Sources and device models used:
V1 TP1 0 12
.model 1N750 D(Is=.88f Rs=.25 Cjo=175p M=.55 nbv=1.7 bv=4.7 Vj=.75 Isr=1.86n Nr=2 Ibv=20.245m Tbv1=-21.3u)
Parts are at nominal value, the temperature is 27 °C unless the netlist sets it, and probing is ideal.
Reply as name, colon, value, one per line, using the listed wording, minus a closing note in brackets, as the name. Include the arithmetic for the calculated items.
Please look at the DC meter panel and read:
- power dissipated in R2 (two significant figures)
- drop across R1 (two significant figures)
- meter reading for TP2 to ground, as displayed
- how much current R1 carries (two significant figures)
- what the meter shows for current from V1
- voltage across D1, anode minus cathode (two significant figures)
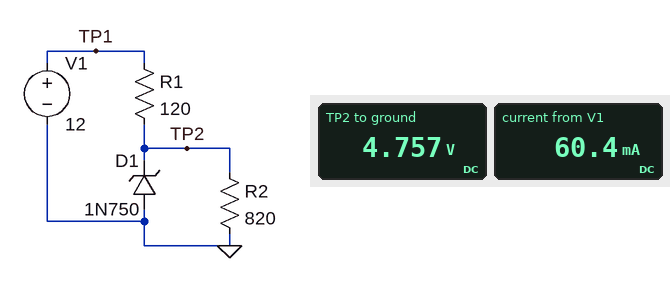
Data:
power dissipated in R2: (4.757 V)^2 / 820 Ω = 28 mW
drop across R1: 12 V - 4.757 V = 7.2 V
meter reading for TP2 to ground, as displayed: 4.757 V
how much current R1 carries: (12 V - 4.757 V) / 120 Ω = 60 mA
what the meter shows for current from V1: 60.4 mA
voltage across D1, anode minus cathode: 0 V - 4.757 V = -4.8 V
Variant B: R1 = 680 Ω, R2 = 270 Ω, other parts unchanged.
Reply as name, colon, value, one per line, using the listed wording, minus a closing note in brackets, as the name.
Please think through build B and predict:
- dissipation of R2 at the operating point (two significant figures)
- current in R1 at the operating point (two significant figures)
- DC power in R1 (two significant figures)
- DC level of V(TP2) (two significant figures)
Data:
dissipation of R2 at the operating point: 43 mW
current in R1 at the operating point: 13 mA
DC power in R1: 110 mW
DC level of V(TP2): 3.4 V
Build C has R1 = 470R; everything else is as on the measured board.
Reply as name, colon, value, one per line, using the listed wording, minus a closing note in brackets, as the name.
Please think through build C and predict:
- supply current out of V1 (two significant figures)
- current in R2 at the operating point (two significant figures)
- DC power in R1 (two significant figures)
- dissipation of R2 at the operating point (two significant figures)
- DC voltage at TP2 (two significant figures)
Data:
supply current out of V1: 16 mA
current in R2 at the operating point: 5.7 mA
DC power in R1: 110 mW
dissipation of R2 at the operating point: 27 mW
DC voltage at TP2: 4.7 V
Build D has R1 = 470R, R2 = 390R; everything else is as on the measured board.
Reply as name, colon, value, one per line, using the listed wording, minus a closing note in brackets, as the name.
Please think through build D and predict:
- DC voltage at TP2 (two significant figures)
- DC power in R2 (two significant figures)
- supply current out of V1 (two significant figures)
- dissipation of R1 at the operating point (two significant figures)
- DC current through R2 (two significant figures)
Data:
DC voltage at TP2: 4.6 V
DC power in R2: 55 mW
supply current out of V1: 16 mA
dissipation of R1 at the operating point: 120 mW
DC current through R2: 12 mA
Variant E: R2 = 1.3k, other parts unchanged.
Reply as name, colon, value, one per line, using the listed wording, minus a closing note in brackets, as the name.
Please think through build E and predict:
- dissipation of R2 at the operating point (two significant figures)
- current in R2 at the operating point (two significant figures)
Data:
dissipation of R2 at the operating point: 17 mW
current in R2 at the operating point: 3.7 mA
